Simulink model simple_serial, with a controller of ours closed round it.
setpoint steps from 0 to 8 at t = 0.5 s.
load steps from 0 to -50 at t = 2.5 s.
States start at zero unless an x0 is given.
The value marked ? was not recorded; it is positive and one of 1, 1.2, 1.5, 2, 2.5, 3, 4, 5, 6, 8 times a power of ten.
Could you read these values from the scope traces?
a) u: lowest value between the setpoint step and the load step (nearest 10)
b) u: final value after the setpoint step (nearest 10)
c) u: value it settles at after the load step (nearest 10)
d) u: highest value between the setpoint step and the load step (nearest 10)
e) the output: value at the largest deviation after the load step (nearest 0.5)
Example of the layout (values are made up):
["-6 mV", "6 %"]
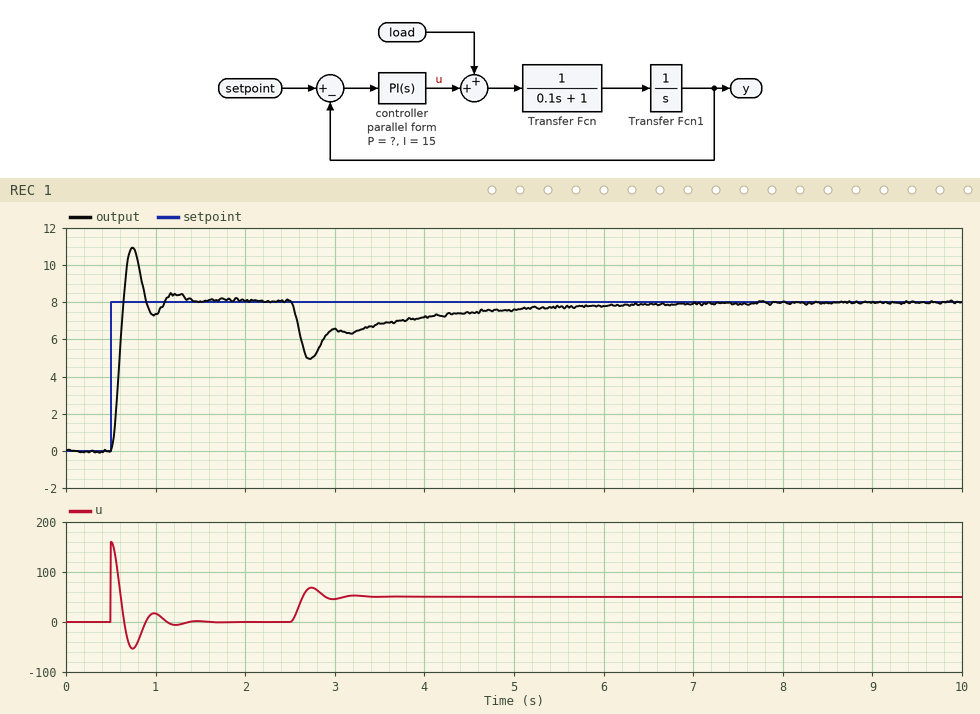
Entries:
["-50", "0", "50", "160", "5.0"]
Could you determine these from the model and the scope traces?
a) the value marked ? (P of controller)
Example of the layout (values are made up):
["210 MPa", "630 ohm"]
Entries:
["20"]
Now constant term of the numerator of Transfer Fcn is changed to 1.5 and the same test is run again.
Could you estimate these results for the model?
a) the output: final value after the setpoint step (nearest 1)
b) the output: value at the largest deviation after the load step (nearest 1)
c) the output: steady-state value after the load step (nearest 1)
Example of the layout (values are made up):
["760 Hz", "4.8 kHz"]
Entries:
["8", "5", "8"]
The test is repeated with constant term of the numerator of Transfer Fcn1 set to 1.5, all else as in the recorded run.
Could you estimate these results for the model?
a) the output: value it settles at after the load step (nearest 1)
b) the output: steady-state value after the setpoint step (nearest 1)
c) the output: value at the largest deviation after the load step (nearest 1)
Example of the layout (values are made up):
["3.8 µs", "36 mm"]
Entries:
["8", "8", "5"]
